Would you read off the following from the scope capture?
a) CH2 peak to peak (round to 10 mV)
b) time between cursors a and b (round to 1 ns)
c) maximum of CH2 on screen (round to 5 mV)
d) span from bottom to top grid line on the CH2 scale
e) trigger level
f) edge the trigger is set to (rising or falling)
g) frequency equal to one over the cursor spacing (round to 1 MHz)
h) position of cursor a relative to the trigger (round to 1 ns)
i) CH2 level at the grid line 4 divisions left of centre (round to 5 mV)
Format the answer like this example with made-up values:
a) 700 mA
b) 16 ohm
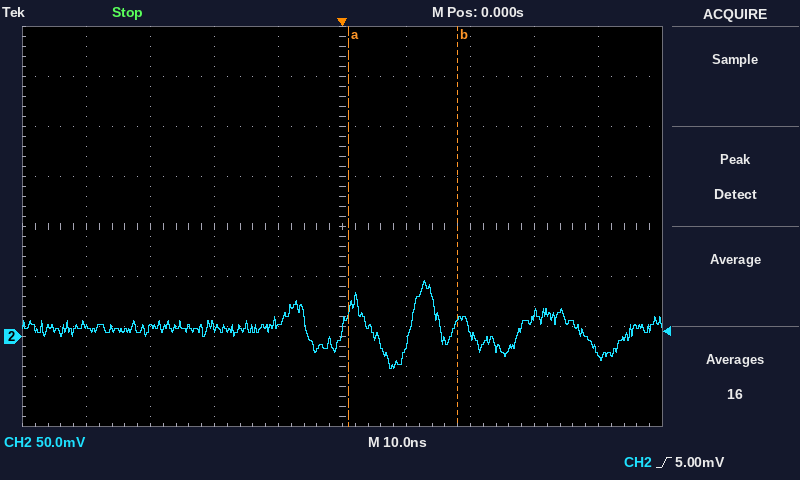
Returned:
a) 90 mV
b) 17 ns
c) 55 mV
d) 400 mV
e) 5.00 mV
f) rising
g) 59 MHz
h) +1 ns
i) 10 mV
